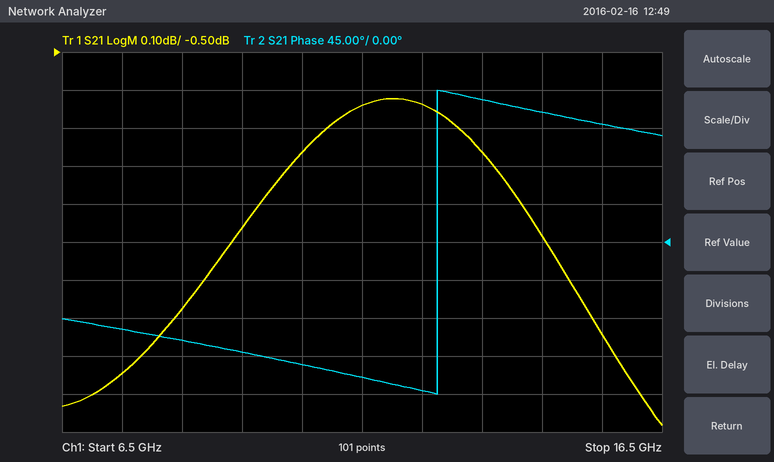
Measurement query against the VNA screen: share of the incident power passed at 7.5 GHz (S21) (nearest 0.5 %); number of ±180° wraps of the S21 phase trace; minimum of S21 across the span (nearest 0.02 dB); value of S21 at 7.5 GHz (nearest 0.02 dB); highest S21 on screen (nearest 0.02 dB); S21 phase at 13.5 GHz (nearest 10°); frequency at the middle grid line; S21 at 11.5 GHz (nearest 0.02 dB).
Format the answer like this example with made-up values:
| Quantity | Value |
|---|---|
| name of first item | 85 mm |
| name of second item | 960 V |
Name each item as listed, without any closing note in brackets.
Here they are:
| Quantity | Value |
|---|---|
| share of the incident power passed at 7.5 GHz (S21) | 73.5 % |
| number of ±180° wraps of the S21 phase trace | 1 |
| minimum of S21 across the span | -1.48 dB |
| value of S21 at 7.5 GHz | -1.34 dB |
| highest S21 on screen | -0.62 dB |
| S21 phase at 13.5 GHz | 170° |
| frequency at the middle grid line | 11.5 GHz |
| S21 at 11.5 GHz | -0.64 dB |
